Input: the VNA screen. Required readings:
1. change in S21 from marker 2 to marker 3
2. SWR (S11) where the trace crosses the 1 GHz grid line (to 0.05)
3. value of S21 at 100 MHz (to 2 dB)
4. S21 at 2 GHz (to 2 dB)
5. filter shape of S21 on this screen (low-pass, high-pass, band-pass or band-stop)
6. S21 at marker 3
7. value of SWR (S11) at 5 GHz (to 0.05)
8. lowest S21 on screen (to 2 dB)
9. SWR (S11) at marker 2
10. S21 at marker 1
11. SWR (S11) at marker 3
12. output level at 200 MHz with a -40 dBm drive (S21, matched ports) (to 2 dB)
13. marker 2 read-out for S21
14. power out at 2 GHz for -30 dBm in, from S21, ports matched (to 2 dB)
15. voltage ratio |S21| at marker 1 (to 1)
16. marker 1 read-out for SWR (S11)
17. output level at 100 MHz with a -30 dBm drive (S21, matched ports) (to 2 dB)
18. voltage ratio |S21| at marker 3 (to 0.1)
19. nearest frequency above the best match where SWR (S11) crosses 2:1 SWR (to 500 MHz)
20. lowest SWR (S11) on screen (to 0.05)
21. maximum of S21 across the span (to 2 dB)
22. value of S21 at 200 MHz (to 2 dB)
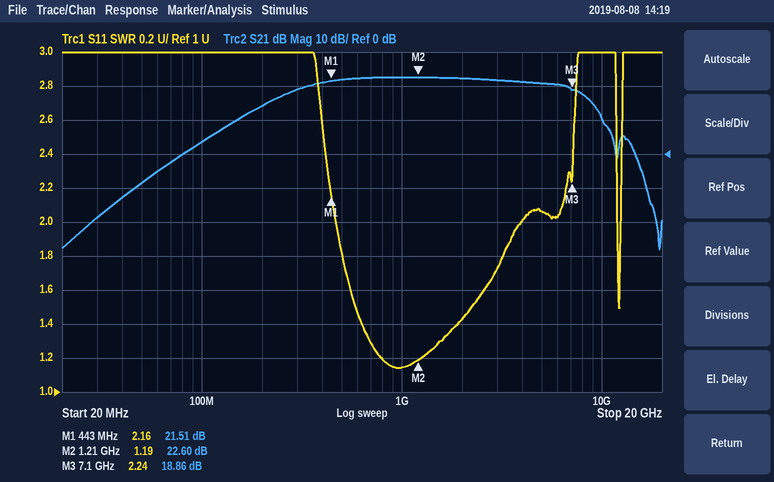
-3.74 dB
1.15
4 dB
22 dB
band-pass
18.86 dB
2.05
-28 dB
1.19
21.51 dB
2.24
-26 dBm
22.60 dB
-8 dBm
12
2.16
-26 dBm
8.8
4.0 GHz
1.15
22 dB
14 dB
